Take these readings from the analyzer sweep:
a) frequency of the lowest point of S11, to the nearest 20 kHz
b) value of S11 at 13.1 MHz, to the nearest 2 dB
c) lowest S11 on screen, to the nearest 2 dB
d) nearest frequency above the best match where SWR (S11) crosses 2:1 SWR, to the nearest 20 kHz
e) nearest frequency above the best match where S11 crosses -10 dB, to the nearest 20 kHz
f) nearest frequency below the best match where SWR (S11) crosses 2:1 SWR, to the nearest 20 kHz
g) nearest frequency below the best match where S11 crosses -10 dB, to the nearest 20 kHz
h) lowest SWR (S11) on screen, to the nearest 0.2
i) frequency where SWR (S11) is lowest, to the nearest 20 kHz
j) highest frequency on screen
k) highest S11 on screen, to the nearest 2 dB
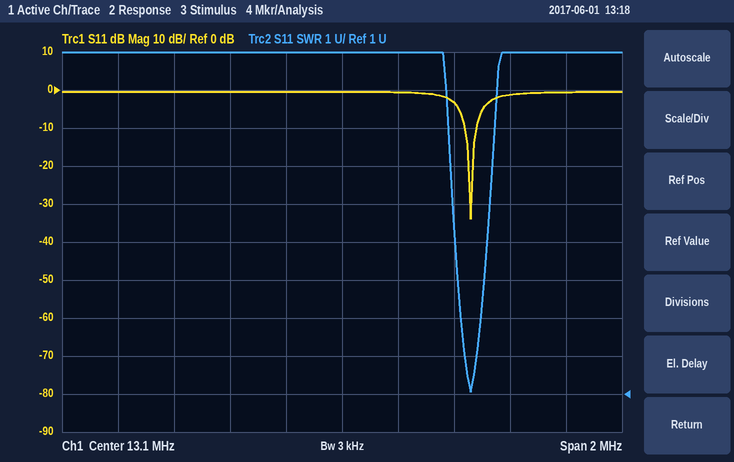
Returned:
13.56 MHz
0 dB
-34 dB
13.58 MHz
13.58 MHz
13.54 MHz
13.54 MHz
1.0
13.56 MHz
14.1 MHz
0 dB
